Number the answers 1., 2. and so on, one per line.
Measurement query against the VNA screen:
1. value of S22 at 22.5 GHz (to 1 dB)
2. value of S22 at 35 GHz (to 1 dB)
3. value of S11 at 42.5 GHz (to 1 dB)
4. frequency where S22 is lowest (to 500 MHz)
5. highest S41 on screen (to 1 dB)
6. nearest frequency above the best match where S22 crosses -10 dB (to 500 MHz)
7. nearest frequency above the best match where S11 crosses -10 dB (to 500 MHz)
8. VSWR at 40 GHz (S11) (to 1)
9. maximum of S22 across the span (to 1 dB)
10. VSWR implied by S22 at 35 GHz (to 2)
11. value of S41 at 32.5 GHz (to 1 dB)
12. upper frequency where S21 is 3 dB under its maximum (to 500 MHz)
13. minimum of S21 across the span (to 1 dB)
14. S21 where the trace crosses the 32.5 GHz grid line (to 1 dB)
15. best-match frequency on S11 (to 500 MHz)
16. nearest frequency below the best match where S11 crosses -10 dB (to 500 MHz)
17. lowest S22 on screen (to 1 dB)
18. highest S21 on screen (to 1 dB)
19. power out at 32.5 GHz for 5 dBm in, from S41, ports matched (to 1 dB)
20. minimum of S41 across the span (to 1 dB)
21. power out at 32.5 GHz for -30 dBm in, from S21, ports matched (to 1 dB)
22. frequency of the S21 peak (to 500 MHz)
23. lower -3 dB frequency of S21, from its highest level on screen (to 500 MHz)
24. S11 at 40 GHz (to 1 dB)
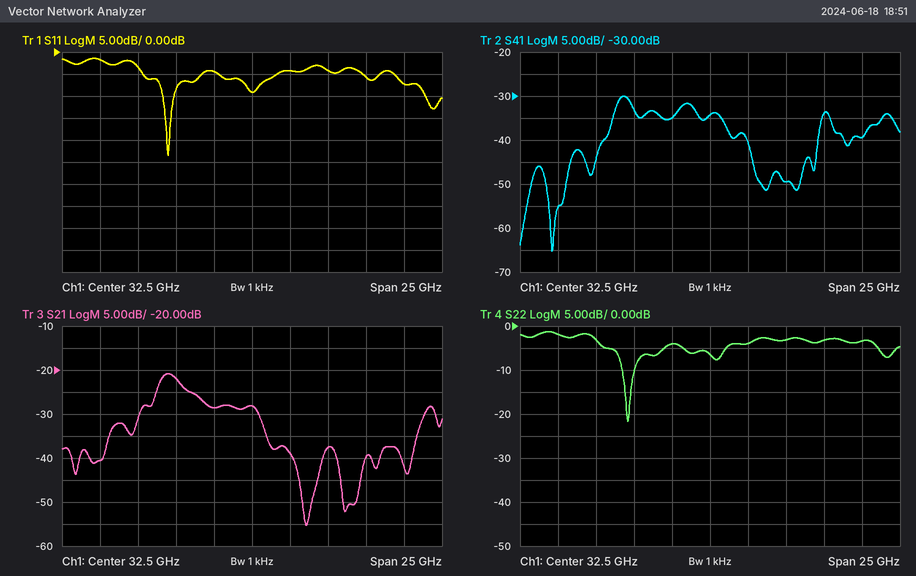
1. -2 dB
2. -4 dB
3. -7 dB
4. 27.0 GHz
5. -30 dB
6. 27.5 GHz
7. 27.5 GHz
8. 3
9. -1 dB
10. 4
11. -34 dB
12. 28.0 GHz
13. -55 dB
14. -28 dB
15. 27.0 GHz
16. 26.5 GHz
17. -22 dB
18. -21 dB
19. -29 dBm
20. -65 dB
21. -58 dBm
22. 27.0 GHz
23. 26.5 GHz
24. -6 dB
